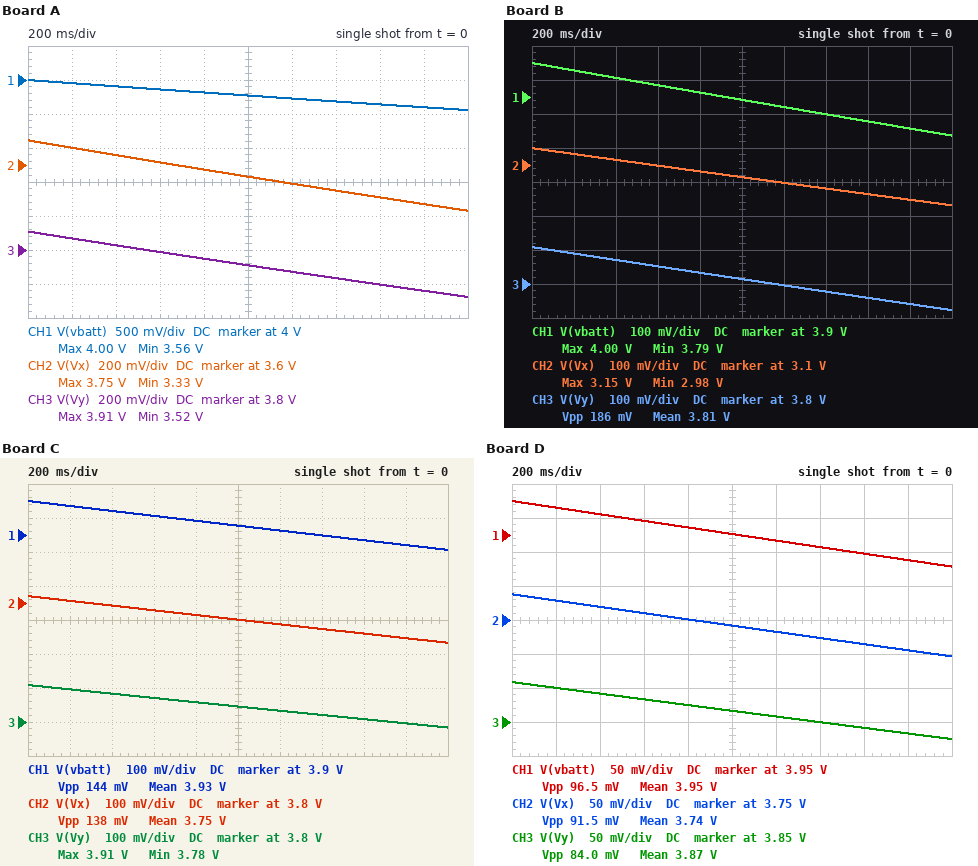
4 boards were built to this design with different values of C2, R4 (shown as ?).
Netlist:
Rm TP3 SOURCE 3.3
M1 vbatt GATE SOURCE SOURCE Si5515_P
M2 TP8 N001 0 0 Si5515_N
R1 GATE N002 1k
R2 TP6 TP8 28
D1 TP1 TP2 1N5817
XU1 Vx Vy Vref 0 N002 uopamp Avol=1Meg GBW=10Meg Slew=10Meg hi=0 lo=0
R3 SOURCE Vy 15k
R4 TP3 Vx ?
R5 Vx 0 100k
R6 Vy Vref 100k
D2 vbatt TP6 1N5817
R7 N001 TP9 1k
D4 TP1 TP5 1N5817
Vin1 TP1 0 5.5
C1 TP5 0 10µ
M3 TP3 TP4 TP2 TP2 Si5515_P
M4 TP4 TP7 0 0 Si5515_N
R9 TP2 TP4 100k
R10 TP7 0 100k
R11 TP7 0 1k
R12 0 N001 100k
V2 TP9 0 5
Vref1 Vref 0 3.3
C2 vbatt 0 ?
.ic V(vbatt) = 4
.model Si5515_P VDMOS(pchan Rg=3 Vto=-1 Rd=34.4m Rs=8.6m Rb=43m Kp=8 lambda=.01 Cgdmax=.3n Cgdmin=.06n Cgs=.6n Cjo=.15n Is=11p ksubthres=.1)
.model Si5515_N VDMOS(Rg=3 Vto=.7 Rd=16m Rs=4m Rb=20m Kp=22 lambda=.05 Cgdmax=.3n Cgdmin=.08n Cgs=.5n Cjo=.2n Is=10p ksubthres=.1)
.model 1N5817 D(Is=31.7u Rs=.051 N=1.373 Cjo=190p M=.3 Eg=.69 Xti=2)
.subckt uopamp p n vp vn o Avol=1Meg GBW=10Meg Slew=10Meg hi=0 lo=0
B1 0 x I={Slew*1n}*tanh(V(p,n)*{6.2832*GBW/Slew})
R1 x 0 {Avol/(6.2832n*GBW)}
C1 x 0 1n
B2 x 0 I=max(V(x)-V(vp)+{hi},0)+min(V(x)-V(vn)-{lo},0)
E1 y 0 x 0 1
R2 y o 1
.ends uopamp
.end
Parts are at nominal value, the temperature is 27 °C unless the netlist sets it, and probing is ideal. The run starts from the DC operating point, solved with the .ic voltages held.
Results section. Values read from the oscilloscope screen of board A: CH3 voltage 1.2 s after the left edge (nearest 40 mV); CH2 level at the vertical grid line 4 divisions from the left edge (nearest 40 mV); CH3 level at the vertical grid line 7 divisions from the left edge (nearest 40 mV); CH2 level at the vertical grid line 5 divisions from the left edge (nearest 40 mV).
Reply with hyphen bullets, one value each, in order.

- 3.68 V
- 3.56 V
- 3.64 V
- 3.52 V
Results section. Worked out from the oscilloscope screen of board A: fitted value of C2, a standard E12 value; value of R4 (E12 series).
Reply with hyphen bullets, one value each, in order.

- 560 mF
- 6.8 kΩ
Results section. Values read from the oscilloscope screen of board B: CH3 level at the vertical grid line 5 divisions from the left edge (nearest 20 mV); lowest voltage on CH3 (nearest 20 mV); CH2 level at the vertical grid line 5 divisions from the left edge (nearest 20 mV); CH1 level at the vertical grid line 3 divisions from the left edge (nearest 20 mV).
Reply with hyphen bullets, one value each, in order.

- 3.82 V
- 3.72 V
- 3.06 V
- 3.94 V
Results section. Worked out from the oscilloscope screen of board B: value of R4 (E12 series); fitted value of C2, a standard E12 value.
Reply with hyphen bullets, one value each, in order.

- 27 kΩ
- 1.2 F
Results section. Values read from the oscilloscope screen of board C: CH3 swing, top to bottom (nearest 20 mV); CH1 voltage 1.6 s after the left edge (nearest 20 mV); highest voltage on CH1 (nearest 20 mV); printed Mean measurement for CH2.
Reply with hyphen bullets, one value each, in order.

- 120 mV
- 3.88 V
- 4.00 V
- 3.75 V
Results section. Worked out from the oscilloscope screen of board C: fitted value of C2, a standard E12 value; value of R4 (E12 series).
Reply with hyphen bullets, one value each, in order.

- 1.8 F
- 4.7 kΩ
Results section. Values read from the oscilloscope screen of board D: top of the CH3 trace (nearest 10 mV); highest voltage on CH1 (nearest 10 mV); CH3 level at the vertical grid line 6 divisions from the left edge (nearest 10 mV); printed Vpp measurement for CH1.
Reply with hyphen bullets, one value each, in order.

- 3.91 V
- 4.00 V
- 3.86 V
- 96.5 mV
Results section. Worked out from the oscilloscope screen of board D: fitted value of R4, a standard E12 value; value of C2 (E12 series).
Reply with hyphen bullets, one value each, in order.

- 5.6 kΩ
- 2.7 F
